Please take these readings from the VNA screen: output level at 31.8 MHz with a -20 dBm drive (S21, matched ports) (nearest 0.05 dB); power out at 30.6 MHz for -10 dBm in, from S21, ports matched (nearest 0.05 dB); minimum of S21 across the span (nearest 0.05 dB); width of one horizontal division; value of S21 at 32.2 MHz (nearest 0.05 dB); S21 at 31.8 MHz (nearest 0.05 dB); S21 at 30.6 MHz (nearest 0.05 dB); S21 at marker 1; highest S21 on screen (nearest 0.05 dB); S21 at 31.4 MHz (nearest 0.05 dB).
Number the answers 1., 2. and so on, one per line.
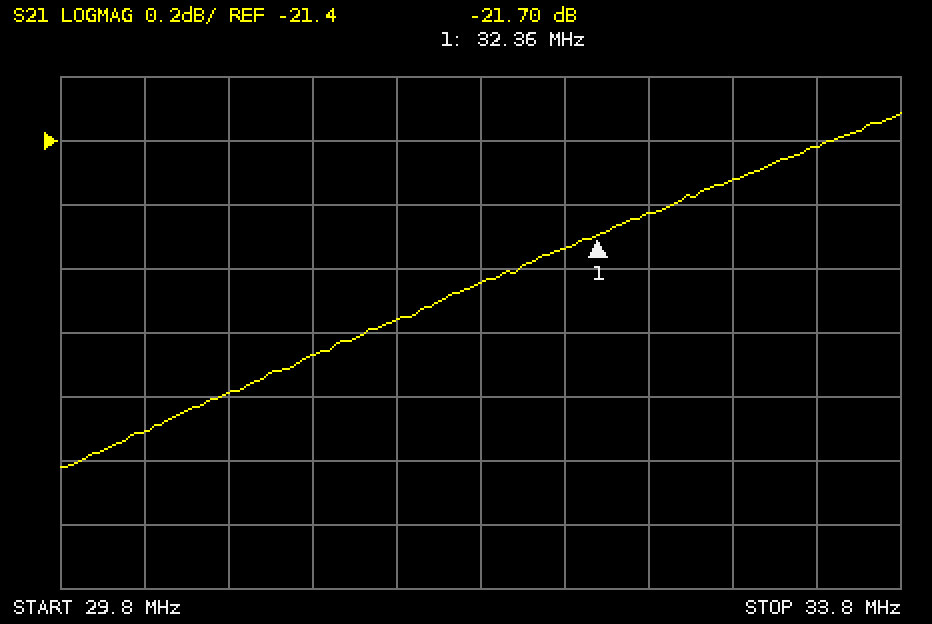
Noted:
1. -41.85 dBm
2. -32.20 dBm
3. -22.40 dB
4. 400 kHz
5. -21.75 dB
6. -21.85 dB
7. -22.20 dB
8. -21.70 dB
9. -21.30 dB
10. -21.95 dB
